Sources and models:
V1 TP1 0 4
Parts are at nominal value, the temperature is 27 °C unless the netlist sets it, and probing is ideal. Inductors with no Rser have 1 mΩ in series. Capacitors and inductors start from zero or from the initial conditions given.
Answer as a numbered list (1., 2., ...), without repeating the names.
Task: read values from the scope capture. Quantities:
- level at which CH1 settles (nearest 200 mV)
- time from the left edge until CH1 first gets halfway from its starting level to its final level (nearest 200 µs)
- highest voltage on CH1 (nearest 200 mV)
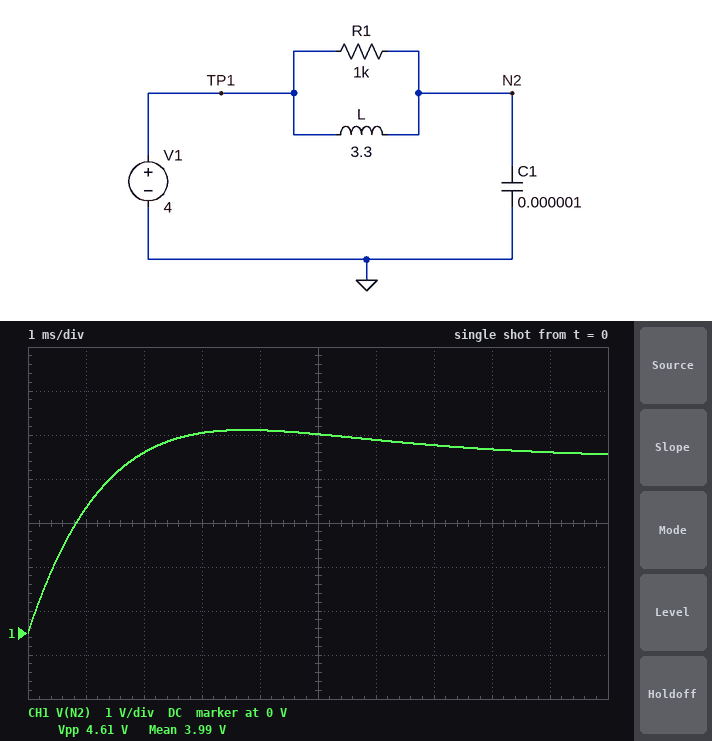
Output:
1. 4.0 V
2. 600 µs
3. 4.6 V
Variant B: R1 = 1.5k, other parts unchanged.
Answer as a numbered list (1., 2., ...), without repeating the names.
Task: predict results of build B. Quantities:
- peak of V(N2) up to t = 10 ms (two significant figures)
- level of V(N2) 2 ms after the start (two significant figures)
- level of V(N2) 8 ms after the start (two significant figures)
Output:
1. 5.0 V
2. 3.9 V
3. 4.2 V
